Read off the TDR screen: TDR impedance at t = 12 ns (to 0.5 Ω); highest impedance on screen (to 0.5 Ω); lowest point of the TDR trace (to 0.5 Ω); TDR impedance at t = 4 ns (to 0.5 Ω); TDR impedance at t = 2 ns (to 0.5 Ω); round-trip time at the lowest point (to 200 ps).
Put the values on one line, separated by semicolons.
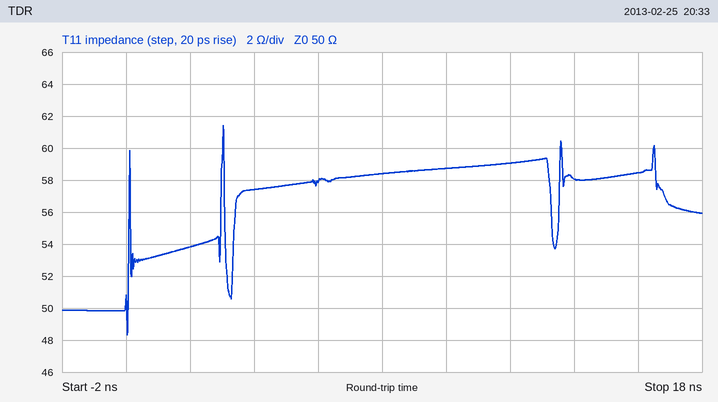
59.0 Ω; 61.5 Ω; 48.5 Ω; 57.5 Ω; 54.0 Ω; 0.0 ns
